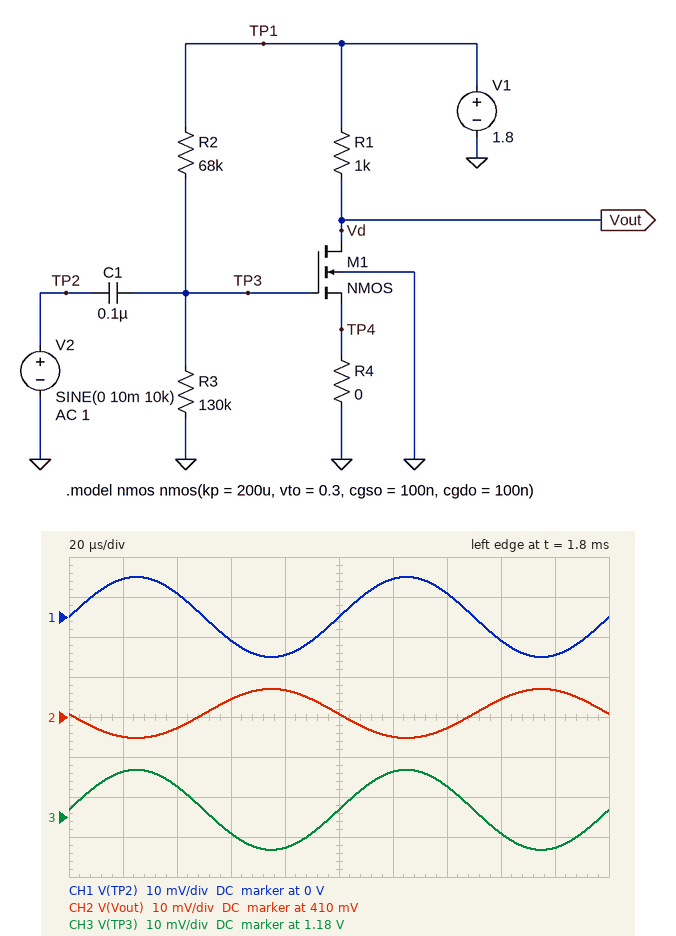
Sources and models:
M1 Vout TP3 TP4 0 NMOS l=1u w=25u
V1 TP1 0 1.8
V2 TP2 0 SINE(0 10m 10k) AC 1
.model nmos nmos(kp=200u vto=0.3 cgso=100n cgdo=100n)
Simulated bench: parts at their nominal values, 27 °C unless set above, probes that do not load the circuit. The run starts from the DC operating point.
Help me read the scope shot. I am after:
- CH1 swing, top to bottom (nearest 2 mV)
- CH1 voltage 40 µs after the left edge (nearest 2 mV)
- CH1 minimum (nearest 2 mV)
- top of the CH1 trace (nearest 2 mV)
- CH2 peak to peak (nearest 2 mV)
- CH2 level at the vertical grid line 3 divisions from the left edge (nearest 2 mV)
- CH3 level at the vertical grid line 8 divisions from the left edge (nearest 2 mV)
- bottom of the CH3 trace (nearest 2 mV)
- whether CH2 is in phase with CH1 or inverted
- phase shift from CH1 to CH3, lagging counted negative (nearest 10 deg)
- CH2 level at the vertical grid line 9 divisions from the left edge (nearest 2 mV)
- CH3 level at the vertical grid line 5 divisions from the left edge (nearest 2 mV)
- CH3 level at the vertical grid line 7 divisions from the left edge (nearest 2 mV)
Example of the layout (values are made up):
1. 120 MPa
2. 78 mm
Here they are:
1. 20 mV
2. 6 mV
3. -10 mV
4. 10 mV
5. 12 mV
6. 414 mV
7. 1.176 V
8. 1.172 V
9. inverted
10. 0 deg
11. 416 mV
12. 1.182 V
13. 1.188 V
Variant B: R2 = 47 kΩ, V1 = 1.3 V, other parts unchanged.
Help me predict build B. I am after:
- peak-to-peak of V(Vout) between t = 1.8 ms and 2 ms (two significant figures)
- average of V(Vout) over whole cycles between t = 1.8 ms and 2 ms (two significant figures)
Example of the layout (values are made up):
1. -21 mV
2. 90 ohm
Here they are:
1. 17 mV
2. 400 mV
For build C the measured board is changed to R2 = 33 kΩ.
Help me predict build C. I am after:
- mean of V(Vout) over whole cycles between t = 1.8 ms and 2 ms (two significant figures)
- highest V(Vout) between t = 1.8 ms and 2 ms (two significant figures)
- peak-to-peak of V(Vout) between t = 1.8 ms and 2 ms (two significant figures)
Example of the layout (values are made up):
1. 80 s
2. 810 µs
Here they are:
1. 300 mV
2. 310 mV
3. 5.9 mV
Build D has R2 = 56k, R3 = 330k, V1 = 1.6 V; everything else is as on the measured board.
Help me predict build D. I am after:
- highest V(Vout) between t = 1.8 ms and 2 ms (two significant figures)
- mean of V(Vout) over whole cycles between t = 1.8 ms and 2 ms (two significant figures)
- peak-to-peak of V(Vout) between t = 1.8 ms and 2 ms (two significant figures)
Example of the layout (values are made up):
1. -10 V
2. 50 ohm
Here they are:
1. 290 mV
2. 280 mV
3. 5.8 mV
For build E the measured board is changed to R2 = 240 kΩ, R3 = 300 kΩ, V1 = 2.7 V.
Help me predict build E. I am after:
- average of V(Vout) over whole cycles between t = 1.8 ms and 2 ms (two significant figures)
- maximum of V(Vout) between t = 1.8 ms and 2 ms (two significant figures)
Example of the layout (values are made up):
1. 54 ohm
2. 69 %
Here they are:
1. 460 mV
2. 470 mV
